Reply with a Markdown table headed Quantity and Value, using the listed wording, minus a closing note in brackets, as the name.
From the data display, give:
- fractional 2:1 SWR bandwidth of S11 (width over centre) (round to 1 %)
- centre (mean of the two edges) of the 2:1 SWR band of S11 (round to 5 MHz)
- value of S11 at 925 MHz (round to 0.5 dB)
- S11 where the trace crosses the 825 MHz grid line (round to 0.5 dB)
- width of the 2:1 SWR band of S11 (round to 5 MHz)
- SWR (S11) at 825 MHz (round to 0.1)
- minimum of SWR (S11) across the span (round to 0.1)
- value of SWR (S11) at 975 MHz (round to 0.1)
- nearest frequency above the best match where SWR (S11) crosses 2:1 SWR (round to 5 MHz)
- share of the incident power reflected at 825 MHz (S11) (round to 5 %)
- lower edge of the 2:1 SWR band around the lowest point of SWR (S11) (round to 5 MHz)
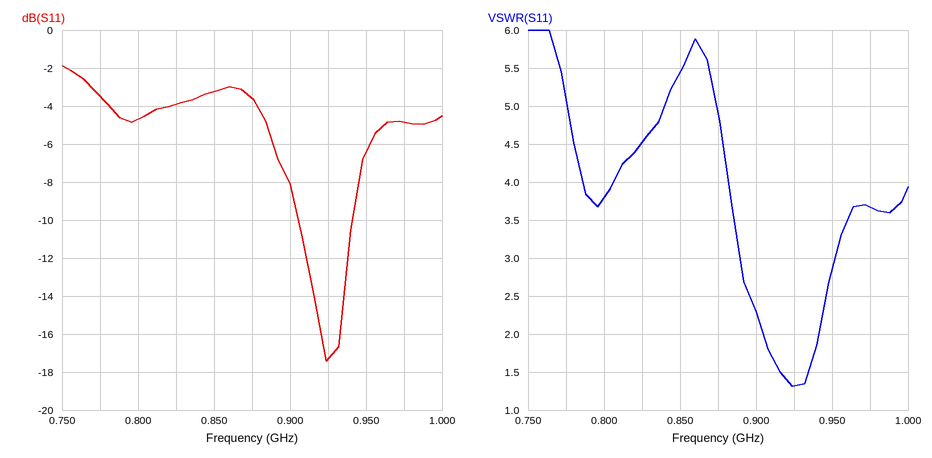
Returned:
| Quantity | Value |
|---|---|
| fractional 2:1 SWR bandwidth of S11 (width over centre) | 4 % |
| centre (mean of the two edges) of the 2:1 SWR band of S11 | 925 MHz |
| value of S11 at 925 MHz | -17.5 dB |
| S11 where the trace crosses the 825 MHz grid line | -4.0 dB |
| width of the 2:1 SWR band of S11 | 35 MHz |
| SWR (S11) at 825 MHz | 4.5 |
| minimum of SWR (S11) across the span | 1.3 |
| value of SWR (S11) at 975 MHz | 3.7 |
| nearest frequency above the best match where SWR (S11) crosses 2:1 SWR | 940 MHz |
| share of the incident power reflected at 825 MHz (S11) | 40 % |
| lower edge of the 2:1 SWR band around the lowest point of SWR (S11) | 905 MHz |
